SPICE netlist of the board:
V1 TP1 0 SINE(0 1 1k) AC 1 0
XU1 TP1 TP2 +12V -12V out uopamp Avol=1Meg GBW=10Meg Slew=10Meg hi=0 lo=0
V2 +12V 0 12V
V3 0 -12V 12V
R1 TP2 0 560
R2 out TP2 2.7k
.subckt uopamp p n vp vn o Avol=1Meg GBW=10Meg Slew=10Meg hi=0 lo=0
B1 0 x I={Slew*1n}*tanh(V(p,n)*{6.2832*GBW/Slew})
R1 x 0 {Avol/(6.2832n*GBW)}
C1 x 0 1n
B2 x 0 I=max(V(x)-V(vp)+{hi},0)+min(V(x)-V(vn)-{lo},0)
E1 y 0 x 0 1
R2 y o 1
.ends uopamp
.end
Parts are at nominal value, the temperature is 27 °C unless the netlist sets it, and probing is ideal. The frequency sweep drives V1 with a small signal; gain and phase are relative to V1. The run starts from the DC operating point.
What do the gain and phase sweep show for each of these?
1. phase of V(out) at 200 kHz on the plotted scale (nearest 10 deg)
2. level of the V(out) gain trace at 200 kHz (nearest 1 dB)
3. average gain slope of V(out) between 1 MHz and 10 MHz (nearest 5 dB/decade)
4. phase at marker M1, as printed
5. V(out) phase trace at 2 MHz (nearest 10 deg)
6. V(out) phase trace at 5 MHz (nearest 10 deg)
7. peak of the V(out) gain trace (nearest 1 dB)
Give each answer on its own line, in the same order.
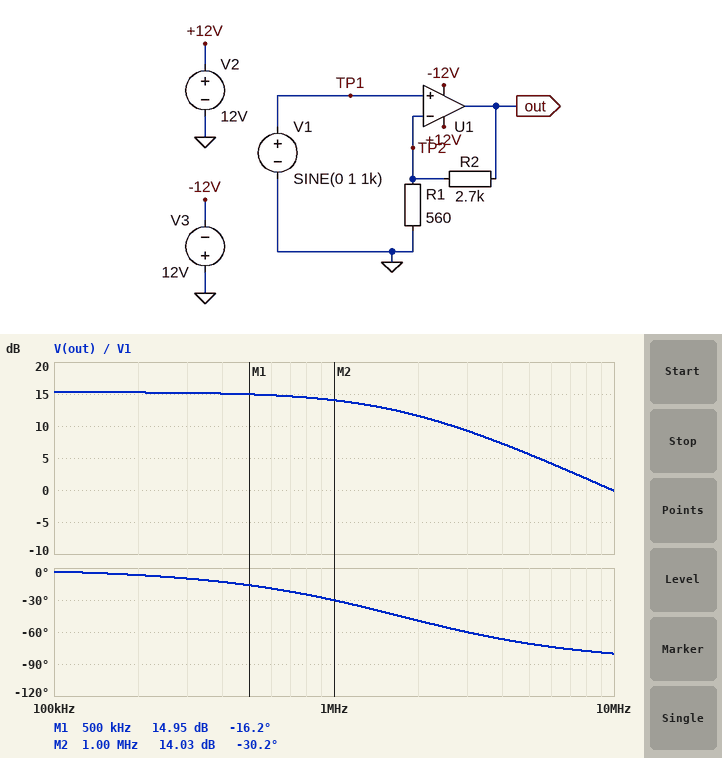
-10 deg
15 dB
-15 dB/decade
-16.2 deg
-50 deg
-70 deg
15 dB
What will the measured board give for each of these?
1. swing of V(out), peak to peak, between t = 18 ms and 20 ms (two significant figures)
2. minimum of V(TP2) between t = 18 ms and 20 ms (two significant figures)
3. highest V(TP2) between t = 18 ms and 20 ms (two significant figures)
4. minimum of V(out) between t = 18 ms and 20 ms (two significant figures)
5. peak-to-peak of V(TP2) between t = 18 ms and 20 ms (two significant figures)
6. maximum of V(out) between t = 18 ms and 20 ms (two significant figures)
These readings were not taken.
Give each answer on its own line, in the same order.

12 V
-1.0 V
1.0 V
-5.8 V
2.0 V
5.8 V
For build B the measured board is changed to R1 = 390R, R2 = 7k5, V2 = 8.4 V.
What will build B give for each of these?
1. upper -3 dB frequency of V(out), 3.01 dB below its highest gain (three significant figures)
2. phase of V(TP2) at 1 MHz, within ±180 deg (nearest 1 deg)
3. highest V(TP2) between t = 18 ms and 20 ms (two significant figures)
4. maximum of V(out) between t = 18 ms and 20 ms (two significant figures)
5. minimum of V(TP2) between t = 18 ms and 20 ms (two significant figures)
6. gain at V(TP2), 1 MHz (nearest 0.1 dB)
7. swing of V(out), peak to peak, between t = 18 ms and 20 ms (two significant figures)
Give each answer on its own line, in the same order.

494 kHz
-64 deg
420 mV
8.4 V
-590 mV
-7.1 dB
20 V
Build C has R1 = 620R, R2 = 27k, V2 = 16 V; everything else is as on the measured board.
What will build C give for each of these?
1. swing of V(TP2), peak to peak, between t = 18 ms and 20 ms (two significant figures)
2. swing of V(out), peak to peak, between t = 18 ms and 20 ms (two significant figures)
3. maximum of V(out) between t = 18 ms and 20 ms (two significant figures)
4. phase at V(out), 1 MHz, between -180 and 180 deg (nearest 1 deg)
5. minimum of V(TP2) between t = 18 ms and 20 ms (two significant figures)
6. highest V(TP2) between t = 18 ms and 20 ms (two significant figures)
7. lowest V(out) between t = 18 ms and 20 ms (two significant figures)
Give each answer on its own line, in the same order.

630 mV
28 V
16 V
-77 deg
-270 mV
360 mV
-12 V
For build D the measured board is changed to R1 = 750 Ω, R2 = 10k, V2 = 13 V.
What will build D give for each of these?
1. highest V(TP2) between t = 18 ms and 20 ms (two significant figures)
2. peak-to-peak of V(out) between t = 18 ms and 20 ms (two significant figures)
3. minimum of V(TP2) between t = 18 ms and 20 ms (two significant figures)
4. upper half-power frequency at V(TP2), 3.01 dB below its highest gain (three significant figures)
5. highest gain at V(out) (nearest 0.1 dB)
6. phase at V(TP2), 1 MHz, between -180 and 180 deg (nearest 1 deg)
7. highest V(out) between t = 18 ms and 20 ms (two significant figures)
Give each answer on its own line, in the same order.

910 mV
25 V
-840 mV
698 kHz
23.1 dB
-55 deg
13 V
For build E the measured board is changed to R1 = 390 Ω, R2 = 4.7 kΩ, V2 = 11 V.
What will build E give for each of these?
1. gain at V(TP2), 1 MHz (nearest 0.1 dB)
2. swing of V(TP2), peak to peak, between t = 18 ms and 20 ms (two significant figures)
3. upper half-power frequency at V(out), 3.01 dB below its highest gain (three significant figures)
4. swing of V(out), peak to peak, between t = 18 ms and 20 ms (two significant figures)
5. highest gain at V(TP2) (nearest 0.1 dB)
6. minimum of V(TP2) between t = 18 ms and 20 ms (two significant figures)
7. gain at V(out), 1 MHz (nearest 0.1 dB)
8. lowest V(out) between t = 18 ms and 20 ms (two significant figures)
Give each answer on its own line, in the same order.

-4.3 dB
1.8 V
766 kHz
23 V
0 dB
-920 mV
18.0 dB
-12 V
